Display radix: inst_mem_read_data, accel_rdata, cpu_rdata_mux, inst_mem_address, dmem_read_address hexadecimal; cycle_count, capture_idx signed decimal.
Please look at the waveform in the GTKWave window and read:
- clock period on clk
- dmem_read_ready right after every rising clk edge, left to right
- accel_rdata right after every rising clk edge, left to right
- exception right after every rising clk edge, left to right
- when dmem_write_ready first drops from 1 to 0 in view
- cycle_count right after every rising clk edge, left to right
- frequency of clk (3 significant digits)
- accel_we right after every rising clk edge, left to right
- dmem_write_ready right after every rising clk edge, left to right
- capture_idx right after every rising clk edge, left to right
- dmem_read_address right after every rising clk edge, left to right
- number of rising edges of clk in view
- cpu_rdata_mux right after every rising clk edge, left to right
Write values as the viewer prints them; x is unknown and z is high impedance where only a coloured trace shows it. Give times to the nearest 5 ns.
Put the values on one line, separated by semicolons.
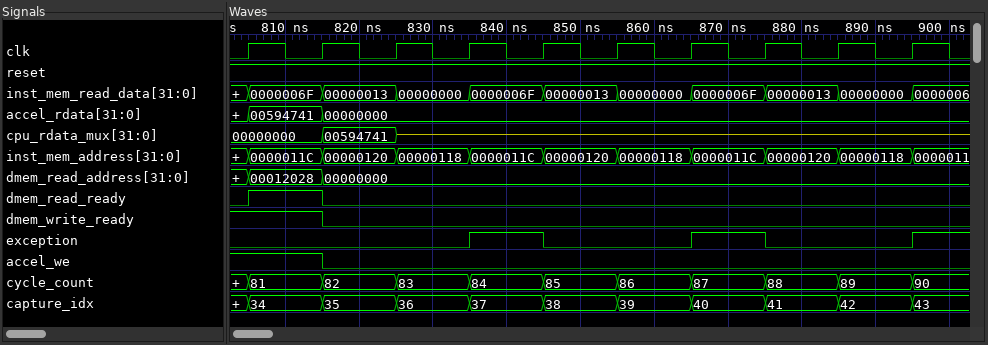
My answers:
10 ns; 1 0 0 0 0 0 0 0 0 0; 00594741, 00000000, 00000000, 00000000, 00000000, 00000000, 00000000, 00000000, 00000000, 00000000; 0 0 0 1 0 0 1 0 0 1; 815 ns; 81, 82, 83, 84, 85, 86, 87, 88, 89, 90; 100 MHz; 1 0 0 0 0 0 0 0 0 0; 1 0 0 0 0 0 0 0 0 0; 34, 35, 36, 37, 38, 39, 40, 41, 42, 43; 00012028, 00000000, 00000000, 00000000, 00000000, 00000000, 00000000, 00000000, 00000000, 00000000; 10; 00000000, 00594741, z, z, z, z, z, z, z, z
